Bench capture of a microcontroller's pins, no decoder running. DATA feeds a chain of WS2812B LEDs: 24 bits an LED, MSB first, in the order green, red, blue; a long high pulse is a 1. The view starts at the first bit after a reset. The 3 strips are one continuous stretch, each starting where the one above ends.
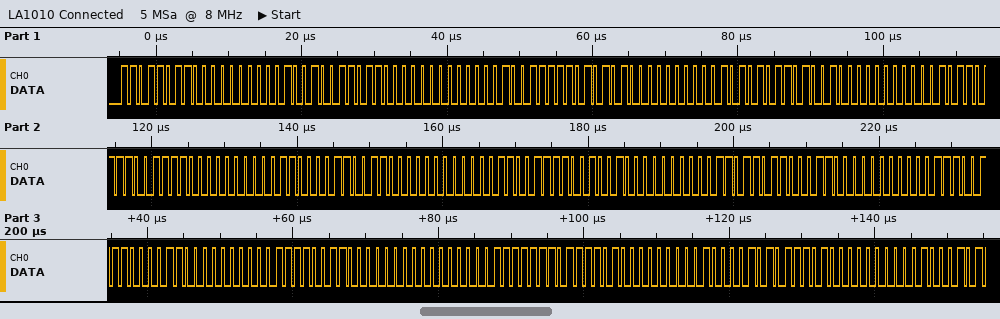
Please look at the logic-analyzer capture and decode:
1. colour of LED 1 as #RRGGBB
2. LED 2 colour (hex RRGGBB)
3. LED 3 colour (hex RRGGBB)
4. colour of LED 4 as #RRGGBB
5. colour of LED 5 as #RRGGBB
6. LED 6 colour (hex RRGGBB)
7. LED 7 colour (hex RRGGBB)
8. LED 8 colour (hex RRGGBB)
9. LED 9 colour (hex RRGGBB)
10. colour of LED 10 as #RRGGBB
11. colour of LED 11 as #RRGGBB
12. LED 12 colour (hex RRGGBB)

#00DB24
#00D827
#00D52A
#00D22D
#00CF30
#00CC33
#00C936
#00C639
#00C33C
#00C03F
#00BD42
#00BA45
